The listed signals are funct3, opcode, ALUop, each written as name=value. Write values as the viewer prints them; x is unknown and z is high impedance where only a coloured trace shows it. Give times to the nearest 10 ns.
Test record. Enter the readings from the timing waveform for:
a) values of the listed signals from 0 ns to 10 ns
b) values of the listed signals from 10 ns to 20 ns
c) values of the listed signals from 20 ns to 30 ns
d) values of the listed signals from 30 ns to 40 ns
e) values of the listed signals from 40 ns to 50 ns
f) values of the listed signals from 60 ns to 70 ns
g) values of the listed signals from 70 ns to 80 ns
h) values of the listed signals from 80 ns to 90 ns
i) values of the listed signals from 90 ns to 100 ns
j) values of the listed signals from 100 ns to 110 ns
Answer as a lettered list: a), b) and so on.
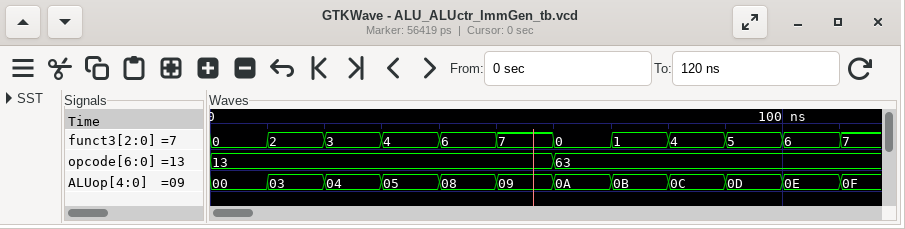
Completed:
a) funct3=0, opcode=13, ALUop=00
b) funct3=2, opcode=13, ALUop=03
c) funct3=3, opcode=13, ALUop=04
d) funct3=4, opcode=13, ALUop=05
e) funct3=6, opcode=13, ALUop=08
f) funct3=0, opcode=63, ALUop=0A
g) funct3=1, opcode=63, ALUop=0B
h) funct3=4, opcode=63, ALUop=0C
i) funct3=5, opcode=63, ALUop=0D
j) funct3=6, opcode=63, ALUop=0E
